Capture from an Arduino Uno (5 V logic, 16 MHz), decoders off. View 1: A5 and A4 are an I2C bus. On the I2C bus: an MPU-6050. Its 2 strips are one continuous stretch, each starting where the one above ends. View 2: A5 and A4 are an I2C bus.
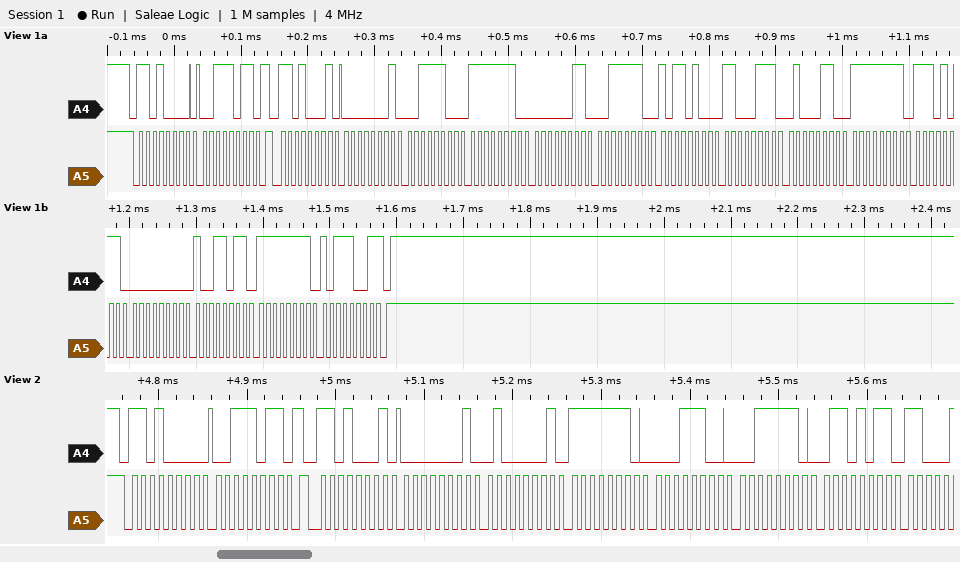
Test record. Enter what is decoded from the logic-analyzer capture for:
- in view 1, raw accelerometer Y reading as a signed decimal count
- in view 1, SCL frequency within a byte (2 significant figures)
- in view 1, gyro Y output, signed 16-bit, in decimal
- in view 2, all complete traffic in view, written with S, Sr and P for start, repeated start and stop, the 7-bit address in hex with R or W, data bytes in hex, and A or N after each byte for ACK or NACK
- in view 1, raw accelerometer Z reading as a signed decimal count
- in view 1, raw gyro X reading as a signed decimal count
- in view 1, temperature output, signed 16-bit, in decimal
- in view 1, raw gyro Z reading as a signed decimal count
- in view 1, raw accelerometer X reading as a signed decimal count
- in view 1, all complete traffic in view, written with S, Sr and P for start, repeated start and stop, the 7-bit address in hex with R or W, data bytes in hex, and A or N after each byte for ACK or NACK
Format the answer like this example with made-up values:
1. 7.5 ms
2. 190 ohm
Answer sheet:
1. -509
2. 100 kHz
3. 155
4. S 68W A 3B A Sr 68R A 01 A 41 A FE A 1C A 3E A 6B A
5. 16052
6. -21
7. -14522
8. -71
9. 316
10. S 68W A 3B A Sr 68R A 01 A 3C A FE A 03 A 3E A B4 A C7 A 46 A FF A EB A 00 A 9B A FF A B9 N P
